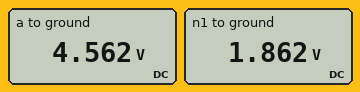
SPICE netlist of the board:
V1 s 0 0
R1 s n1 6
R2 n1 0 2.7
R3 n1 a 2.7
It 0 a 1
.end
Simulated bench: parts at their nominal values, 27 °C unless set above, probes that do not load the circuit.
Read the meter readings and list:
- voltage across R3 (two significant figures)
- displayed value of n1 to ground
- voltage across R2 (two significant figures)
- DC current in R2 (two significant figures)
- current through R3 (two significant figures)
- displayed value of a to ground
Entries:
2.7 V
1.862 V
1.9 V
690 mA
1.0 A
4.562 V
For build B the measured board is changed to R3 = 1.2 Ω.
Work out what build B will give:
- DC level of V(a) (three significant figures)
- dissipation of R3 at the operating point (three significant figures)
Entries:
3.06 V
1.20 W
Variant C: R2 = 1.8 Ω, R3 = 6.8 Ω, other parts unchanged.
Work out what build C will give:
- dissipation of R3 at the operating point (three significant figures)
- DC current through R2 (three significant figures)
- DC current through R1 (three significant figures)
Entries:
6.80 W
769 mA
231 mA
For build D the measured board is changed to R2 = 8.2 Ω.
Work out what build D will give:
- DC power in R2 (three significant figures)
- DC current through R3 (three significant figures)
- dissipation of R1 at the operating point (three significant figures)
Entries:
1.46 W
1.00 A
2.00 W
